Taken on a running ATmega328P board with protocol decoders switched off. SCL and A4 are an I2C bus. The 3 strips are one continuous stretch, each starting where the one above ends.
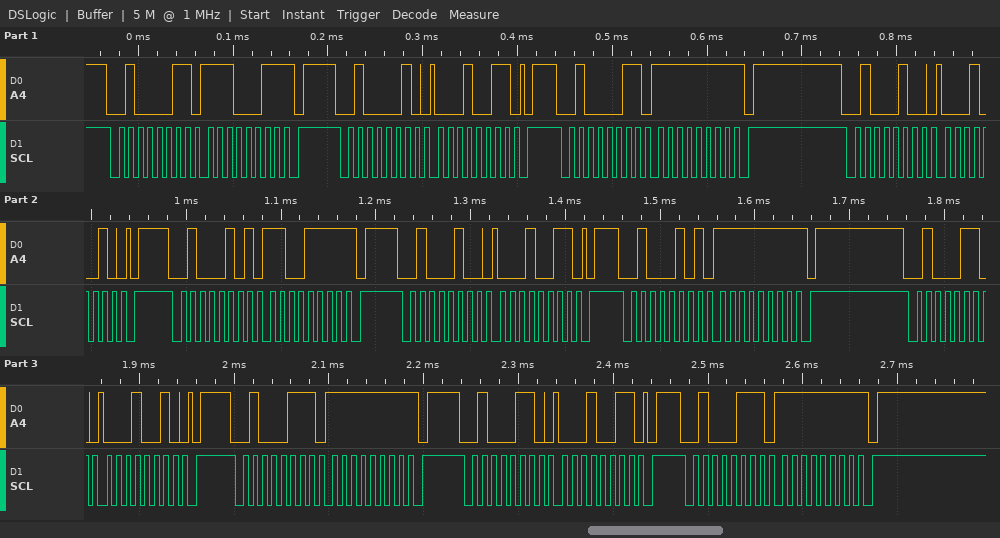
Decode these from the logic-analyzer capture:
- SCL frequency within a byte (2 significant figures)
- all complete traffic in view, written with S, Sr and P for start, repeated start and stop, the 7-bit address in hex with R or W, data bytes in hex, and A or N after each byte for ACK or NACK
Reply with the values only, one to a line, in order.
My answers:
100 kHz
S 21R A E3 N P S 21W A 13 A P S 21R A FF N P S 22W A 12 A P S 22R A CF N P S 22W A 13 A P S 22R A FF N P S 23W A 12 A P S 23R A FF N P S 23W A 13 A P S 23R A FF N P
